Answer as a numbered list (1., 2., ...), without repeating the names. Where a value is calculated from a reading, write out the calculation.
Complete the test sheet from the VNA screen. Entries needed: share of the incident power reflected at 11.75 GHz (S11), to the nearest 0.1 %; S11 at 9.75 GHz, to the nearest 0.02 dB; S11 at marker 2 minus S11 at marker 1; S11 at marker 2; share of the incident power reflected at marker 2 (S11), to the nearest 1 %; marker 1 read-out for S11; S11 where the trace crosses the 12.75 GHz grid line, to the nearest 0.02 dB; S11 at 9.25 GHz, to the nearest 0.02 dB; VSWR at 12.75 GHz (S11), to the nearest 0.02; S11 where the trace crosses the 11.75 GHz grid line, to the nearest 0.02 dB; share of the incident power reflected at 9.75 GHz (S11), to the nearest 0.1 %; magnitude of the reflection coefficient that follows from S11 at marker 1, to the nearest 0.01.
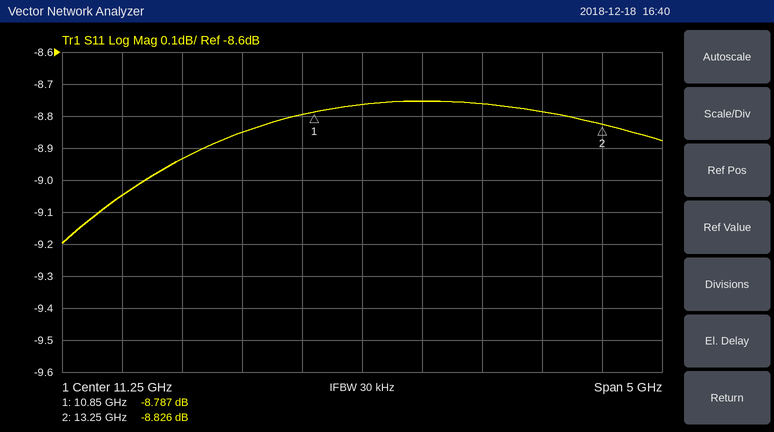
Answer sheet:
1. 10^(-8.76/10) ≈ 13.3 %
2. -8.94 dB
3. -8.826 − (-8.787) = -0.039 dB
4. -8.826 dB
5. 10^(-8.826/10) ≈ 13 %
6. -8.787 dB
7. -8.78 dB
8. -9.04 dB
9. |Γ| = 10^(-8.78/20) = 0.3639; VSWR = (1 + 0.3639)/(1 − 0.3639) ≈ 2.14
10. -8.76 dB
11. 10^(-8.94/10) ≈ 12.8 %
12. 10^(-8.787/20) ≈ 0.36
